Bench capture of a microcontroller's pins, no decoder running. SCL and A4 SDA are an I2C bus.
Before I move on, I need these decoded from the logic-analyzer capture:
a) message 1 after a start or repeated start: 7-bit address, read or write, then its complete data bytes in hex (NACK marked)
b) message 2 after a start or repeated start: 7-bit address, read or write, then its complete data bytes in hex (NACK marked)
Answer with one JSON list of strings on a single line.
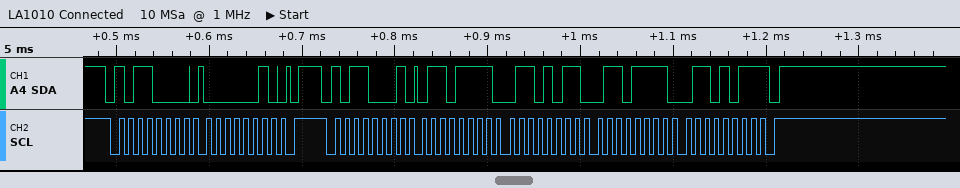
["0x58 write: 02", "0x58 read: 6F 6B 6F 6B NACK"]
